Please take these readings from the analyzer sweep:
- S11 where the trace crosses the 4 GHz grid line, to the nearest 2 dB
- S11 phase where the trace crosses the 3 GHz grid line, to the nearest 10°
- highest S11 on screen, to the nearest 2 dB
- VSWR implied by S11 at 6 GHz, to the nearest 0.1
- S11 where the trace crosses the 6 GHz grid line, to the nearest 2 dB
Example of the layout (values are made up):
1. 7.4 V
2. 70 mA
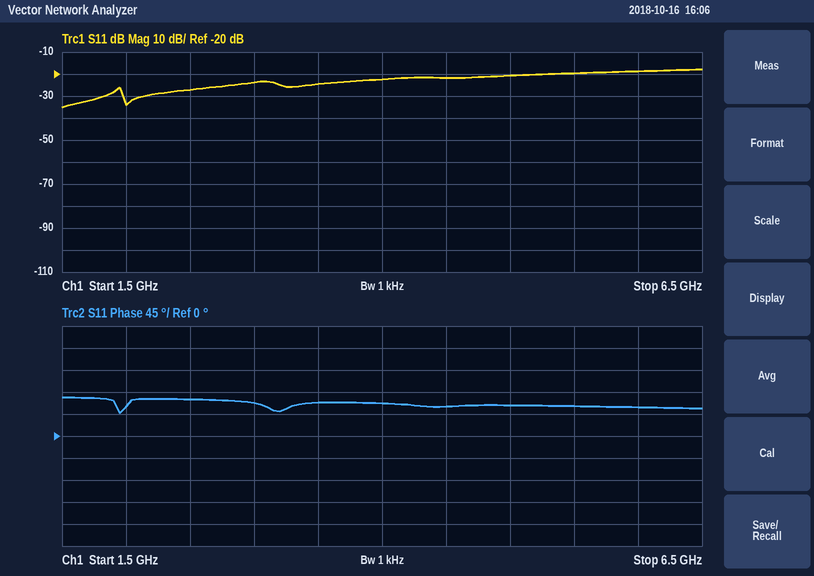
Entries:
1. -22 dB
2. 70°
3. -18 dB
4. 1.3
5. -18 dB
